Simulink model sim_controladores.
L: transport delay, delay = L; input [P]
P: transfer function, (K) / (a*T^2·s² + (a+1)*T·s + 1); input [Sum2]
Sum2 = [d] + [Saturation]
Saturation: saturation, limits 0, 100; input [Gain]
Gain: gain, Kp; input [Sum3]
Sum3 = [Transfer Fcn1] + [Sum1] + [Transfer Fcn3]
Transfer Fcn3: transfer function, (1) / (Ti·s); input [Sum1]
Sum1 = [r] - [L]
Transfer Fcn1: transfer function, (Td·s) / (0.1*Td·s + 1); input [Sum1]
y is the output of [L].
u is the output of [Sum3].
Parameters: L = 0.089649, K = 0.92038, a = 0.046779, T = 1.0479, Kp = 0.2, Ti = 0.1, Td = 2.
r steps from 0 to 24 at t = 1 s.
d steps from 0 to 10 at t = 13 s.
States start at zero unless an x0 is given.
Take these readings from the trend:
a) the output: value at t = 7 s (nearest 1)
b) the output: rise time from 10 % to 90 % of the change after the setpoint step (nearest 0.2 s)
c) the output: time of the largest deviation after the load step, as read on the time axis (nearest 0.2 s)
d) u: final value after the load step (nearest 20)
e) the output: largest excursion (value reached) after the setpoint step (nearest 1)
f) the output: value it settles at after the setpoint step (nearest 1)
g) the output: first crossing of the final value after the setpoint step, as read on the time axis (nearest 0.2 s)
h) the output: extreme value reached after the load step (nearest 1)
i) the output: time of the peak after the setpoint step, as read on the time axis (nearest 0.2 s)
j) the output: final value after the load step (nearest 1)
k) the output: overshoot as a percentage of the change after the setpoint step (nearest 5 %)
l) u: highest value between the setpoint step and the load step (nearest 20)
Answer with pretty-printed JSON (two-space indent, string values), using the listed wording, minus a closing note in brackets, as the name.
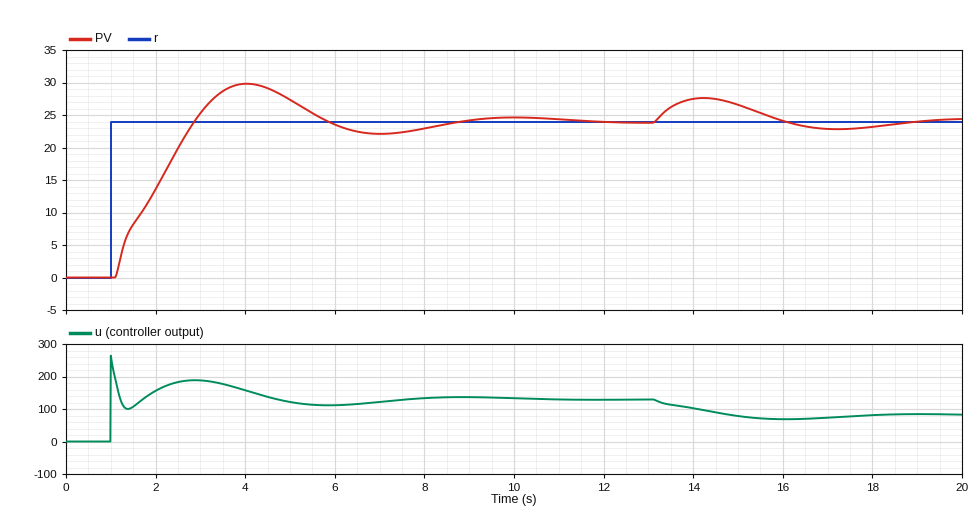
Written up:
{
  "the output: value at t = 7 s": "22",
  "the output: rise time from 10 % to 90 % of the change after the setpoint step": "1.4 s",
  "the output: time of the largest deviation after the load step, as read on the time axis": "14.2 s",
  "u: final value after the load step": "80",
  "the output: largest excursion (value reached) after the setpoint step": "30",
  "the output: value it settles at after the setpoint step": "24",
  "the output: first crossing of the final value after the setpoint step, as read on the time axis": "2.8 s",
  "the output: extreme value reached after the load step": "28",
  "the output: time of the peak after the setpoint step, as read on the time axis": "4.0 s",
  "the output: final value after the load step": "24",
  "the output: overshoot as a percentage of the change after the setpoint step": "25 %",
  "u: highest value between the setpoint step and the load step": "260"
}
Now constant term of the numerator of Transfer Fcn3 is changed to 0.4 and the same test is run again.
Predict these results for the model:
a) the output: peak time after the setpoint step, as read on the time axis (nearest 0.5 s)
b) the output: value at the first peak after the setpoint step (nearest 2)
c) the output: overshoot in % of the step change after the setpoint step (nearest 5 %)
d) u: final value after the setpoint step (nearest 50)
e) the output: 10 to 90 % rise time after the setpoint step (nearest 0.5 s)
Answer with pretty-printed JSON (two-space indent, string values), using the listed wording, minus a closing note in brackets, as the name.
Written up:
{
  "the output: peak time after the setpoint step, as read on the time axis": "6.5 s",
  "the output: value at the first peak after the setpoint step": "26",
  "the output: overshoot in % of the step change after the setpoint step": "10 %",
  "u: final value after the setpoint step": "150",
  "the output: 10 to 90 % rise time after the setpoint step": "3.0 s"
}
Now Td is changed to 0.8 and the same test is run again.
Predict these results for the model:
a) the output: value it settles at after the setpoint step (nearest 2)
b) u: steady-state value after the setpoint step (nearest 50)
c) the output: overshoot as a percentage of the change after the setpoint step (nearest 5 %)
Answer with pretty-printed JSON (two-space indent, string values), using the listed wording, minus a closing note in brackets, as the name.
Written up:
{
  "the output: value it settles at after the setpoint step": "24",
  "u: steady-state value after the setpoint step": "150",
  "the output: overshoot as a percentage of the change after the setpoint step": "30 %"
}
